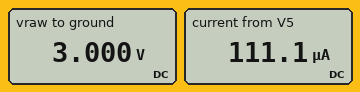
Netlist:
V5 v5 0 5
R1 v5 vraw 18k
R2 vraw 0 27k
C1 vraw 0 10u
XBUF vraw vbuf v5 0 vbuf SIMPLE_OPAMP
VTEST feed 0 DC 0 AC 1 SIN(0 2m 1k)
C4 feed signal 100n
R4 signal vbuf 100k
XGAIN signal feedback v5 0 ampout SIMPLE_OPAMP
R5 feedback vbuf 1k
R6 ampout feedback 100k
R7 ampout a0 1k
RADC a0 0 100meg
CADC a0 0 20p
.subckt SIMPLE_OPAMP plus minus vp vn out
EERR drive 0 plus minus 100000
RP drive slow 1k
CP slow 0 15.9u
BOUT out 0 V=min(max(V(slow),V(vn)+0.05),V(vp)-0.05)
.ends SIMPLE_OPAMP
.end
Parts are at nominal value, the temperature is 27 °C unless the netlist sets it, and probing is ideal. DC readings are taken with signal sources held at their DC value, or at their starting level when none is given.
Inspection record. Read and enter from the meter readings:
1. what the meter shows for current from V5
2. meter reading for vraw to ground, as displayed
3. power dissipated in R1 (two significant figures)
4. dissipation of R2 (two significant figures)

111.1 µA
3.000 V
220 µW
330 µW
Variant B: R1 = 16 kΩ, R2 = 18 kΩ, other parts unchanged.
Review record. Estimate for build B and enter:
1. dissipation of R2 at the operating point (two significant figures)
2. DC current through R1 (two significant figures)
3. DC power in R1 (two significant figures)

390 µW
150 µA
350 µW
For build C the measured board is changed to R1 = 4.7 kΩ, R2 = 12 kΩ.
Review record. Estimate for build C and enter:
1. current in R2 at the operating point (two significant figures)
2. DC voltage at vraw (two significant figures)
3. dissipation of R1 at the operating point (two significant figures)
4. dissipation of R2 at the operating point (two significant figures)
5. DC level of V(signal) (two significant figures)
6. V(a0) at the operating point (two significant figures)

6.1 µA
73 mV
5.2 mW
440 nW
55 mV
50 mV
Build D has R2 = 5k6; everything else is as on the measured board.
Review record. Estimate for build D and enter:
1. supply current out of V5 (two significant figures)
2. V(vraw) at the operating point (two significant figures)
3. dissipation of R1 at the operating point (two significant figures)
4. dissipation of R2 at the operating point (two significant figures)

210 µA
1.2 V
810 µW
250 µW
